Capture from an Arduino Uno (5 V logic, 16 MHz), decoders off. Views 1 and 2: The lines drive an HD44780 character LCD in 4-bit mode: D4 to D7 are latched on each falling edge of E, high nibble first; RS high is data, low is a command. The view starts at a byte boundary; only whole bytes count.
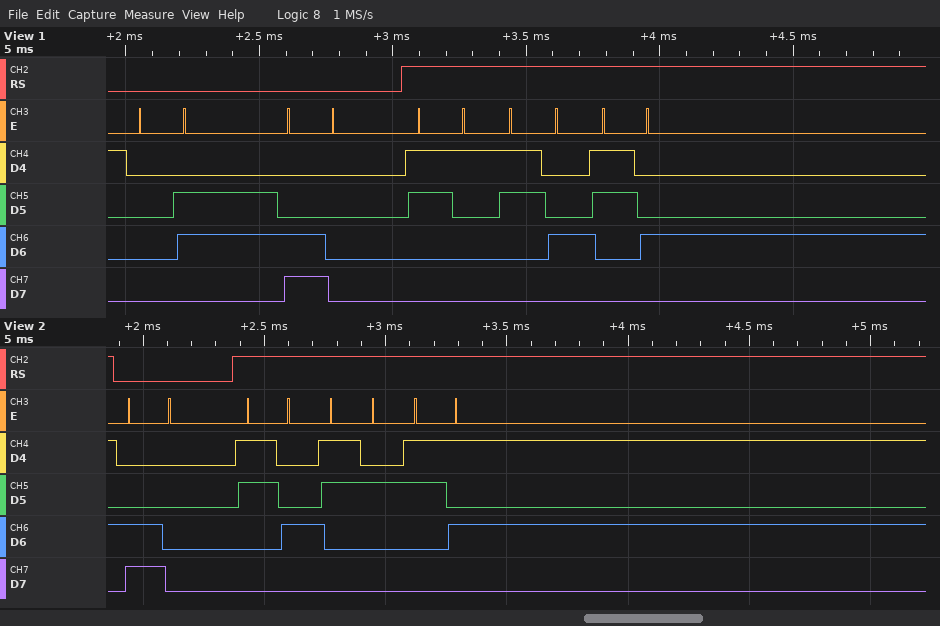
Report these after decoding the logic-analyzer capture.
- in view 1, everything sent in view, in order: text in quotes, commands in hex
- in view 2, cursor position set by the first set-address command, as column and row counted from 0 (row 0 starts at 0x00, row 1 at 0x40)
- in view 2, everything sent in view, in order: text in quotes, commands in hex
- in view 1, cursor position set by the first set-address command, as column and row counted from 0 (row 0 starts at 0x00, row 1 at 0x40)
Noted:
0x06 0xC0 "144"
column 0, row 1
0xC0 "425"
column 0, row 1
